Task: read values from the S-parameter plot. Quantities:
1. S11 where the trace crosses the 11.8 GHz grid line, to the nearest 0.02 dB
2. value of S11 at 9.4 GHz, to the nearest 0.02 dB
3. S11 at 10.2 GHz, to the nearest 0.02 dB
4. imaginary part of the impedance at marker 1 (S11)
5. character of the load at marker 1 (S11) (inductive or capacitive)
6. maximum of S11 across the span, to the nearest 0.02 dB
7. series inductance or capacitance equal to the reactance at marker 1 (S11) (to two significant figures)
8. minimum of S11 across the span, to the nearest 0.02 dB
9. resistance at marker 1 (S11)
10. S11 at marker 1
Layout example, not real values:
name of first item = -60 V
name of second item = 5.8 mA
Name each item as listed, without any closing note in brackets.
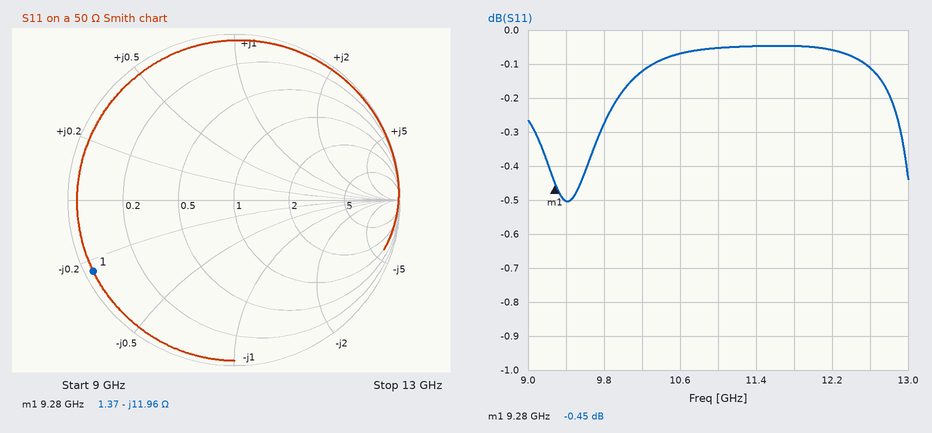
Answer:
S11 where the trace crosses the 11.8 GHz grid line, to the nearest 0.02 dB = -0.04 dB
value of S11 at 9.4 GHz, to the nearest 0.02 dB = -0.50 dB
S11 at 10.2 GHz, to the nearest 0.02 dB = -0.12 dB
imaginary part of the impedance at marker 1 = -11.96 Ω
character of the load at marker 1 (S11) = capacitive
maximum of S11 across the span, to the nearest 0.02 dB = -0.04 dB
series inductance or capacitance equal to the reactance at marker 1 (S11) = 1.4 pF
minimum of S11 across the span, to the nearest 0.02 dB = -0.50 dB
resistance at marker 1 = 1.37 Ω
S11 at marker 1 = -0.45 dB
